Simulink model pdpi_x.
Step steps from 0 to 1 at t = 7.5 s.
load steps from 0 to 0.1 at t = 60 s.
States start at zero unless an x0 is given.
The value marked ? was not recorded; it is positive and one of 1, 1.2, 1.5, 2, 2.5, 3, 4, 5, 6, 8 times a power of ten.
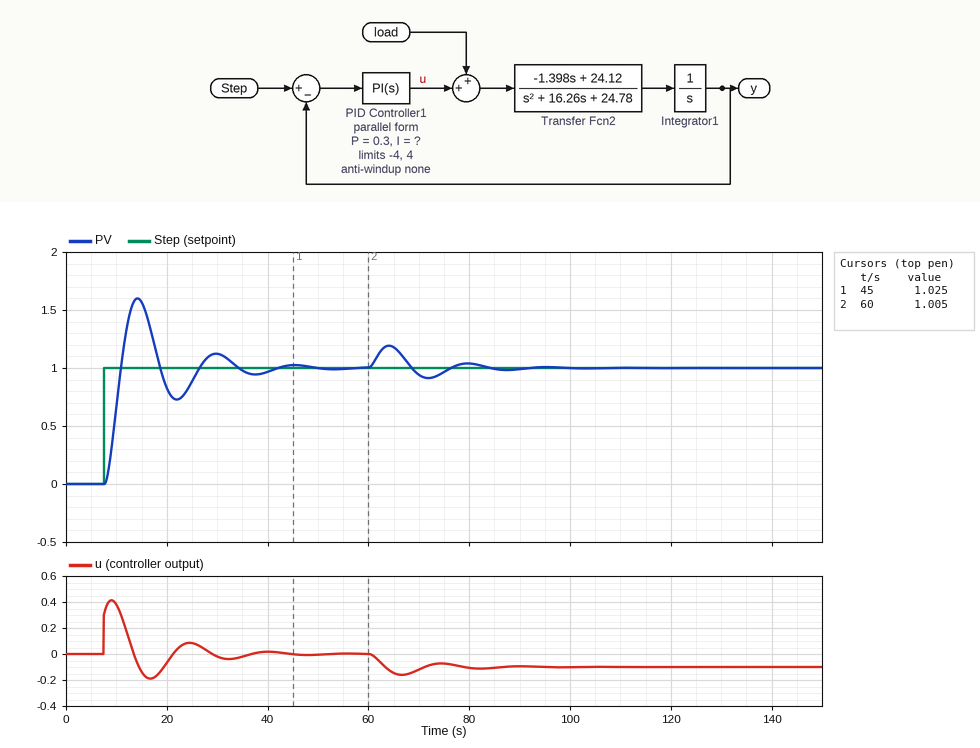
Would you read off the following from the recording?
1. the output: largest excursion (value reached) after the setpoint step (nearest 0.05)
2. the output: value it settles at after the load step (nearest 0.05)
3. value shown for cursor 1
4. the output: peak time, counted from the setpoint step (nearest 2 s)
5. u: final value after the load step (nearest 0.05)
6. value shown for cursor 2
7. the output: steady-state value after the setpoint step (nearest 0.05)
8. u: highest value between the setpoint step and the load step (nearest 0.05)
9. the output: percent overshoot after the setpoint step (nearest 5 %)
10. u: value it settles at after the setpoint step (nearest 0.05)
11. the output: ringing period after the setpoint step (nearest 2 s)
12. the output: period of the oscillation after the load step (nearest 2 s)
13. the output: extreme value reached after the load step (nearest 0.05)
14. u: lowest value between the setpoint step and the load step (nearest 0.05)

1.60
1.00
1.025
6 s
-0.10
1.005
1.00
0.40
60 %
0.00
16 s
16 s
1.20
-0.20
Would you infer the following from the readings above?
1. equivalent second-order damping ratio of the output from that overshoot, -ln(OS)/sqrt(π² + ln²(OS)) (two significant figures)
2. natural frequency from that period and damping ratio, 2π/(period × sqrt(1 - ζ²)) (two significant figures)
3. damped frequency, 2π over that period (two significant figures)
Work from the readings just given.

0.16
0.40 rad/s
0.39 rad/s
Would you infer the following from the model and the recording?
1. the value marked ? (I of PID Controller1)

0.15
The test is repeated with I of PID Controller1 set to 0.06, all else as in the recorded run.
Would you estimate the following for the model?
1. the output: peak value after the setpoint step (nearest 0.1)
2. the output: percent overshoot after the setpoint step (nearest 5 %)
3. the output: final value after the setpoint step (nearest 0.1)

1.3
35 %
1.0
